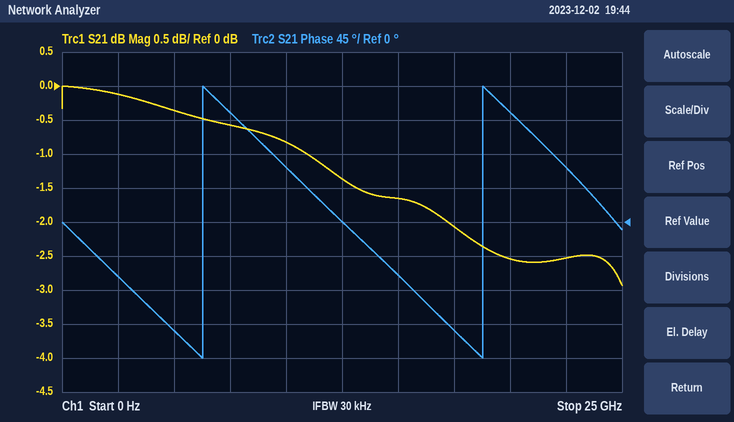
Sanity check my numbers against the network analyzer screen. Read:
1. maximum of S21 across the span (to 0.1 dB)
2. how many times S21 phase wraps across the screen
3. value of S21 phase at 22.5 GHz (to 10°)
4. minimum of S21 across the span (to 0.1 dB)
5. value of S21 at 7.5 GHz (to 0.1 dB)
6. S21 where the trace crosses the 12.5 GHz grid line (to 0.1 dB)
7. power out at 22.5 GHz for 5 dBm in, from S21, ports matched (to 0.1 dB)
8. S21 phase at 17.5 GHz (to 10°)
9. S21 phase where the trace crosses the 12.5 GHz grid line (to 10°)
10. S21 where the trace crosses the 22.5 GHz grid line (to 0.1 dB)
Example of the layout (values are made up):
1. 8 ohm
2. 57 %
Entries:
1. 0.0 dB
2. 2
3. 70°
4. -2.9 dB
5. -0.6 dB
6. -1.4 dB
7. 2.5 dBm
8. -140°
9. 0°
10. -2.5 dB
